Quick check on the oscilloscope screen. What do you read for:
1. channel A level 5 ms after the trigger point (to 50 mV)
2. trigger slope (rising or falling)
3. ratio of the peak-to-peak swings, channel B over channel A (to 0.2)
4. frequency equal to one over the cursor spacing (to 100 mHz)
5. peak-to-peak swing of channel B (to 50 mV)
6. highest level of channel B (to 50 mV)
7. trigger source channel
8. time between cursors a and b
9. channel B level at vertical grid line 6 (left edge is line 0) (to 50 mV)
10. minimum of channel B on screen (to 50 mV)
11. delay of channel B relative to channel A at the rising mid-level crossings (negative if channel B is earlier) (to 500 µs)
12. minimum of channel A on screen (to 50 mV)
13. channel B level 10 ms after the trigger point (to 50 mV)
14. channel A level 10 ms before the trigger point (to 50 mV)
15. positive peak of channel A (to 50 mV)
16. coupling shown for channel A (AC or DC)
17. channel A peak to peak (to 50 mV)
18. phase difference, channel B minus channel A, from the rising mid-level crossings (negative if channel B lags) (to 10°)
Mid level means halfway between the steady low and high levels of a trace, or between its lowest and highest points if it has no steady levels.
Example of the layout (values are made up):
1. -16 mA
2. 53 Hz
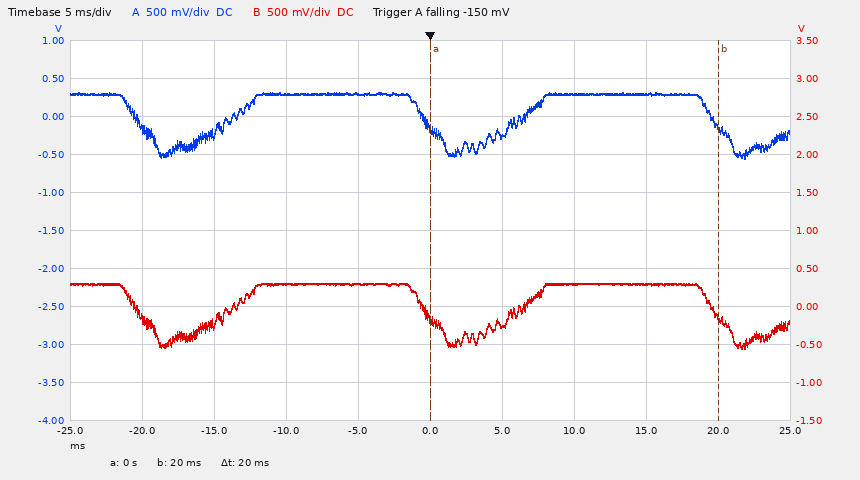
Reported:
1. -250 mV
2. falling
3. 1.0
4. 50.0 Hz
5. 850 mV
6. 300 mV
7. channel A
8. 20 ms
9. -250 mV
10. -550 mV
11. 0.0 ms
12. -550 mV
13. 300 mV
14. 300 mV
15. 300 mV
16. DC
17. 850 mV
18. 0°
